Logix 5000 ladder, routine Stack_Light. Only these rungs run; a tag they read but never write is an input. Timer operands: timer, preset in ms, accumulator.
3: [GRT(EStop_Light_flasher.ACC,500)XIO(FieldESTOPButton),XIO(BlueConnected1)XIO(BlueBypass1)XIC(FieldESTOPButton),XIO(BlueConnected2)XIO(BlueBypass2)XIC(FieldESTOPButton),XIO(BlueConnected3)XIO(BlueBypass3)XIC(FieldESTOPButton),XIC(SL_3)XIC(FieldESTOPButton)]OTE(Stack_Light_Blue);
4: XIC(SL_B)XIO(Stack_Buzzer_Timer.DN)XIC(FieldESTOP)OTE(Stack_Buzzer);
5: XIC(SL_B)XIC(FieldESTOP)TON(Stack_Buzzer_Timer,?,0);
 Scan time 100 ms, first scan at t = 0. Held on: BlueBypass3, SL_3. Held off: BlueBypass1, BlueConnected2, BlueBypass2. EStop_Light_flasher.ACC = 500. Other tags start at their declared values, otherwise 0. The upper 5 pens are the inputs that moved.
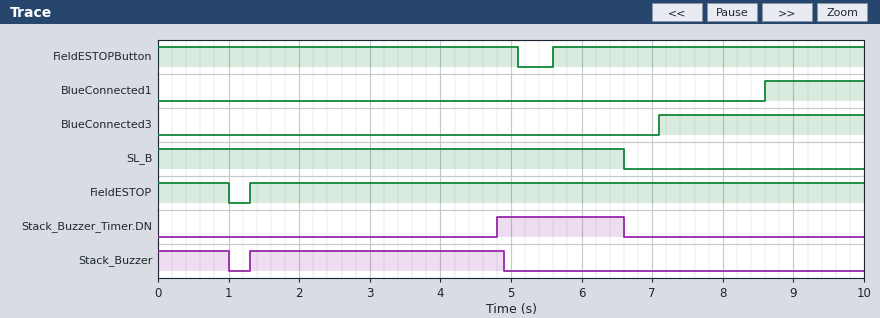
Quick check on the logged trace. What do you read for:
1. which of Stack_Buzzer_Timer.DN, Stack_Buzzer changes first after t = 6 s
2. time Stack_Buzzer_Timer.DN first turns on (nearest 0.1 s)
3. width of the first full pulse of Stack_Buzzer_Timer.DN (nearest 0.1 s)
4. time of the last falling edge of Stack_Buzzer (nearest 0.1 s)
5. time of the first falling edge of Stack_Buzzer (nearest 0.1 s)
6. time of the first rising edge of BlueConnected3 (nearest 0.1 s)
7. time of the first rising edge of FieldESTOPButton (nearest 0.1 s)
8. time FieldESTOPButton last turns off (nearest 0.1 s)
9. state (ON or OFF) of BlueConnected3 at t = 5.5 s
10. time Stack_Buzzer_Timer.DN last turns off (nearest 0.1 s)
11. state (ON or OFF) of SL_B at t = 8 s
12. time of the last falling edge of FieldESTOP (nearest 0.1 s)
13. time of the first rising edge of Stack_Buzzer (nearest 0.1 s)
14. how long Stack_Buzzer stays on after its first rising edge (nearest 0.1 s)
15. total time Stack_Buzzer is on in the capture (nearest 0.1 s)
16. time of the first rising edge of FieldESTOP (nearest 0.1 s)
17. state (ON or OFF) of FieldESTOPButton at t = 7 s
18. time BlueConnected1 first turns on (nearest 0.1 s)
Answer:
Stack_Buzzer_Timer.DN
4.8 s
1.8 s
4.9 s
1.0 s
7.1 s
5.6 s
5.1 s
OFF
6.6 s
OFF
1.0 s
1.3 s
3.6 s
4.6 s
1.3 s
ON
8.6 s
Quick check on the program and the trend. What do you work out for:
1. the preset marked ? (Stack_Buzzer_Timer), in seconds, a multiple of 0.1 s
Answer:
3.5 s
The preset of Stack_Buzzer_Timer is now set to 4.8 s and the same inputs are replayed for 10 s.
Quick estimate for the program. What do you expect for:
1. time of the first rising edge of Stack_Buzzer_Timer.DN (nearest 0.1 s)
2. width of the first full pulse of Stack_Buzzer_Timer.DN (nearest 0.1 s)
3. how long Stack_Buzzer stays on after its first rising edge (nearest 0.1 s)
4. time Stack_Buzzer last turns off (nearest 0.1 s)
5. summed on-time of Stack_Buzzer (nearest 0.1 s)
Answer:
6.1 s
0.5 s
4.9 s
6.2 s
5.9 s
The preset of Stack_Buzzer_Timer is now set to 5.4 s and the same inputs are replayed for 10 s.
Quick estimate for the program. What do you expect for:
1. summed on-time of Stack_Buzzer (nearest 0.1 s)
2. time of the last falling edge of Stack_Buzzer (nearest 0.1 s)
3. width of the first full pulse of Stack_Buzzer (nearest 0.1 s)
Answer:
6.3 s
6.6 s
5.3 s
